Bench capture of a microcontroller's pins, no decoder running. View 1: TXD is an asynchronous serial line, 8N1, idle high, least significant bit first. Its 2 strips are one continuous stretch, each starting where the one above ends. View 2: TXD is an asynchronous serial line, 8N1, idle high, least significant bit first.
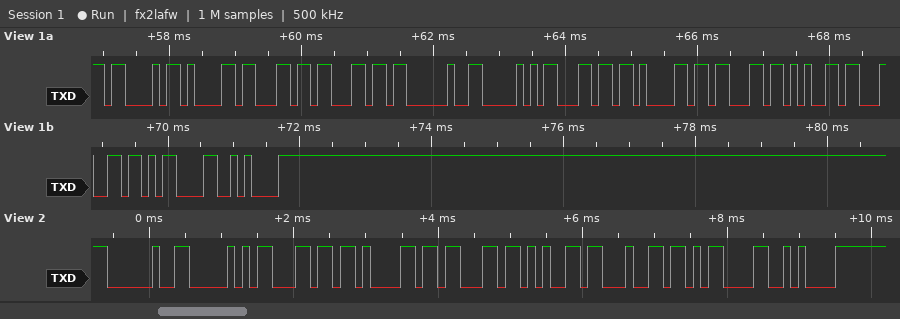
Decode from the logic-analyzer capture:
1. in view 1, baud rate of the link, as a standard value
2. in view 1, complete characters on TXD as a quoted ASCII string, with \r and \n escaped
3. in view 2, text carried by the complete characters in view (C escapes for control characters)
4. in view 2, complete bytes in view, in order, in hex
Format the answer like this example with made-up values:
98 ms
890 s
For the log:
9600 baud
"Call Placed\r\n"
" Placed\r\n"
0x20 0x50 0x6C 0x61 0x63 0x65 0x64 0x0D 0x0A
